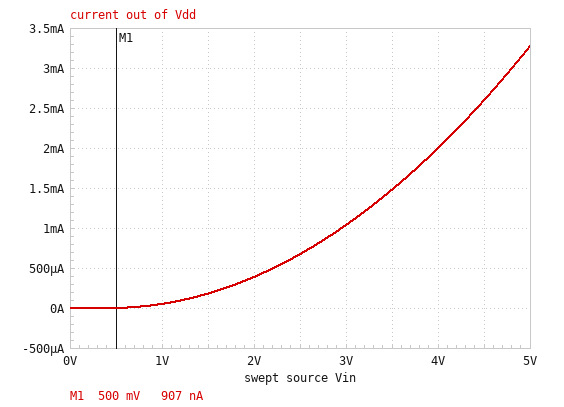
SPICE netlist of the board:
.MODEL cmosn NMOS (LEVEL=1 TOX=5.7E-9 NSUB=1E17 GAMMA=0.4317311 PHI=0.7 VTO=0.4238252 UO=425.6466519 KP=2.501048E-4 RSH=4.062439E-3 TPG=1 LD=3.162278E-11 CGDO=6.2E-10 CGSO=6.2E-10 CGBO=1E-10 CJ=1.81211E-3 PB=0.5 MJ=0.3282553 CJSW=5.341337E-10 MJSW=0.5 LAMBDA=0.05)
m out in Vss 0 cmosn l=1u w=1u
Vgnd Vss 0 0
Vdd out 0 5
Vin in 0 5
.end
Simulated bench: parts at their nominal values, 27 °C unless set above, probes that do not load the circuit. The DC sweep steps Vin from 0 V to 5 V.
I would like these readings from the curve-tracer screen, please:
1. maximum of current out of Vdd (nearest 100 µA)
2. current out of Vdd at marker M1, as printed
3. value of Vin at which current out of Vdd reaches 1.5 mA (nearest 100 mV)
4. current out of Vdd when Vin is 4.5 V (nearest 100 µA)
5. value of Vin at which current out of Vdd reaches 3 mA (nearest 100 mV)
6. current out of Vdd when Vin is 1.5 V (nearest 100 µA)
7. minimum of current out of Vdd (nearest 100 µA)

3.3 mA
907 nA
3.5 V
2.6 mA
4.8 V
200 µA
0 A
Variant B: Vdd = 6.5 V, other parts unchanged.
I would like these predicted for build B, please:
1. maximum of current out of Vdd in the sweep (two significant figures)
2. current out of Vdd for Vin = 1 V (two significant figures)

3.5 mA
55 µA
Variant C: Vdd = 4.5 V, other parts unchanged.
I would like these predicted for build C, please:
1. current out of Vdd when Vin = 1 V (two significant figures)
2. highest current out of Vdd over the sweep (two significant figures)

51 µA
3.2 mA
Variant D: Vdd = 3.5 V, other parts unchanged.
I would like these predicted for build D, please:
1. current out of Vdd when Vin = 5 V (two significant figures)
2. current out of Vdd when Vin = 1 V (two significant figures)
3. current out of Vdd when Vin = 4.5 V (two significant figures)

2.9 mA
49 µA
2.4 mA
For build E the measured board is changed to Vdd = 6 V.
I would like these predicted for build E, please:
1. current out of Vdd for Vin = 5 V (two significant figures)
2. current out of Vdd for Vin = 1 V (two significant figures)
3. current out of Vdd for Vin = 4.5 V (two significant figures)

3.4 mA
54 µA
2.7 mA
